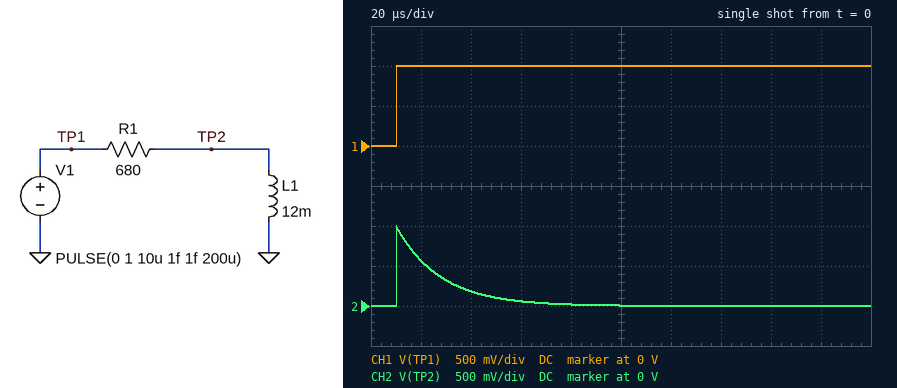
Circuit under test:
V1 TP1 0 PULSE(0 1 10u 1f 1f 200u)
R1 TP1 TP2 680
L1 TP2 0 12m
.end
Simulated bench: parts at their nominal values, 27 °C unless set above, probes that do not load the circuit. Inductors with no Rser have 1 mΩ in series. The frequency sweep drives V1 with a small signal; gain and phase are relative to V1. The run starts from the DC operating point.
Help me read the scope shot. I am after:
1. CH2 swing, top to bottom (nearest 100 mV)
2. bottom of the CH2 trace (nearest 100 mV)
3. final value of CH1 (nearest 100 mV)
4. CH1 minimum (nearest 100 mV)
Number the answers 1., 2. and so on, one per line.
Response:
1. 1.0 V
2. 0 V
3. 1.0 V
4. 0 V
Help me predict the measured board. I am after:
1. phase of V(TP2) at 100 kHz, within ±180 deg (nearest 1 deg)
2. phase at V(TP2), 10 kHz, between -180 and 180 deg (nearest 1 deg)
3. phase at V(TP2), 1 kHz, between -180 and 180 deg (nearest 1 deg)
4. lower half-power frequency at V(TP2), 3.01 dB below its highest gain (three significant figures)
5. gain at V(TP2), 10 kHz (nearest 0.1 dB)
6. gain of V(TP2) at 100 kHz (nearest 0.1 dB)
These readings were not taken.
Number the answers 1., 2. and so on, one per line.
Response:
1. 5 deg
2. 42 deg
3. 84 deg
4. 9.02 kHz
5. -2.6 dB
6. 0 dB
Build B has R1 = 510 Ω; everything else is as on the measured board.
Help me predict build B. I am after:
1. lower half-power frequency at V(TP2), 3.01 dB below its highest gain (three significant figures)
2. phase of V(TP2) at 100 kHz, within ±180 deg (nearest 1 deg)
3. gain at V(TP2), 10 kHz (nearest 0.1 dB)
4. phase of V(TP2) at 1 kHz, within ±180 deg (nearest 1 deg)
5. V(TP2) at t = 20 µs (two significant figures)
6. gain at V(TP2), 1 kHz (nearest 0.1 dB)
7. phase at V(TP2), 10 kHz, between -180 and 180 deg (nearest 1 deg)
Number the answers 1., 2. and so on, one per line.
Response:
1. 6.76 kHz
2. 4 deg
3. -1.6 dB
4. 82 deg
5. 650 mV
6. -16.7 dB
7. 34 deg
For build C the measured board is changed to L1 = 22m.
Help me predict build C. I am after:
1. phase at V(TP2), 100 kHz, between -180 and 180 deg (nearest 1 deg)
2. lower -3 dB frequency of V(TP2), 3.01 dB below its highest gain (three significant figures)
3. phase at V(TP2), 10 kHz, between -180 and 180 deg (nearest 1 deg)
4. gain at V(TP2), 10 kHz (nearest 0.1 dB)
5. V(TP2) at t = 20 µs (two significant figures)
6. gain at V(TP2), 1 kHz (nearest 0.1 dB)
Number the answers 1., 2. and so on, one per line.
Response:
1. 3 deg
2. 4.92 kHz
3. 26 deg
4. -0.9 dB
5. 730 mV
6. -14.0 dB
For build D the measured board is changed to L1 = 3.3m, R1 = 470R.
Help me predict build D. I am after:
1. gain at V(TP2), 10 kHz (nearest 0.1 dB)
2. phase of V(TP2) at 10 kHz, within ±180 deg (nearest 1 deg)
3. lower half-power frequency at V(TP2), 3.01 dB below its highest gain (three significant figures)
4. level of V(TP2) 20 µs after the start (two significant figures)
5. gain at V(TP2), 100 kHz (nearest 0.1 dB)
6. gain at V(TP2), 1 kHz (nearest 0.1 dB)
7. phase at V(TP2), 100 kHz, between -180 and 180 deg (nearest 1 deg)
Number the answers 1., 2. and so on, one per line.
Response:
1. -7.9 dB
2. 66 deg
3. 22.7 kHz
4. 240 mV
5. -0.2 dB
6. -27.1 dB
7. 13 deg
